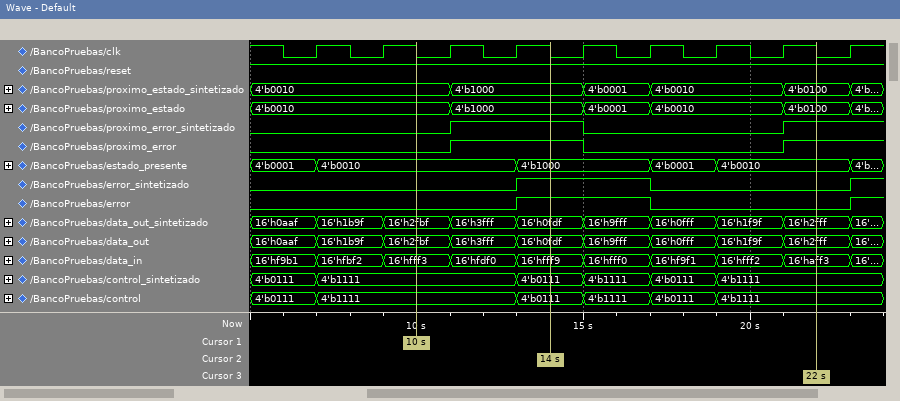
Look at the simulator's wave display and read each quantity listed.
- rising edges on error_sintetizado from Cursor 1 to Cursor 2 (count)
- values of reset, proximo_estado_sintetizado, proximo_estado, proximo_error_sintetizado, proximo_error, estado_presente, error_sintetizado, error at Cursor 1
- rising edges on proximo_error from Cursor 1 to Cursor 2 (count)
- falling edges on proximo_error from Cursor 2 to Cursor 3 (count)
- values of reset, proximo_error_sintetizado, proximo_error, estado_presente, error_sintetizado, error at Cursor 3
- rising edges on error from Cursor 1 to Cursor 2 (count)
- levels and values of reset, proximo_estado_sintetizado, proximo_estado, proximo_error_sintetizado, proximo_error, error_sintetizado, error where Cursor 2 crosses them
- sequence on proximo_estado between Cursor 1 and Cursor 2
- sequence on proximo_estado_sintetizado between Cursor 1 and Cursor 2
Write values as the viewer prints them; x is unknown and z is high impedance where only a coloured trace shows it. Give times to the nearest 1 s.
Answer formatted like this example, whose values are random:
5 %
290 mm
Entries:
1
reset=1, proximo_estado_sintetizado=4'b0010, proximo_estado=4'b0010, proximo_error_sintetizado=0, proximo_error=0, estado_presente=4'b0010, error_sintetizado=0, error=0
1
1
reset=1, proximo_error_sintetizado=1, proximo_error=1, estado_presente=4'b0010, error_sintetizado=0, error=0
1
reset=1, proximo_estado_sintetizado=4'b1000, proximo_estado=4'b1000, proximo_error_sintetizado=1, proximo_error=1, error_sintetizado=1, error=1
4'b0010, 4'b1000
4'b0010, 4'b1000
